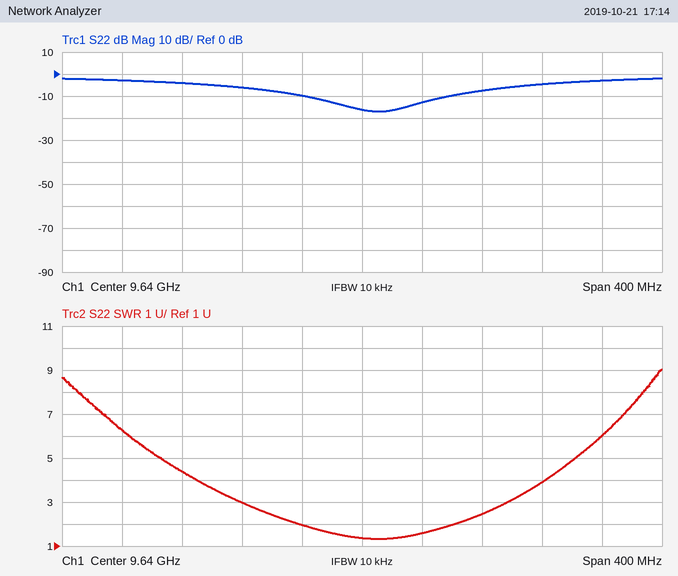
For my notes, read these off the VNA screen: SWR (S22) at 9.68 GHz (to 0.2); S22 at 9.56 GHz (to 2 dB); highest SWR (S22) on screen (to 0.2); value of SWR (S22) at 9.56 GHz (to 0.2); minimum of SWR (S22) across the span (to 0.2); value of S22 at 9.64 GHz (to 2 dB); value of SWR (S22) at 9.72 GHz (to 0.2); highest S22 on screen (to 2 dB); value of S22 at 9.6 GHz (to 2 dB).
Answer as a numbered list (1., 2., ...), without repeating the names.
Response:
1. 1.6
2. -6 dB
3. 9.0
4. 3.0
5. 1.4
6. -16 dB
7. 2.4
8. -2 dB
9. -10 dB
